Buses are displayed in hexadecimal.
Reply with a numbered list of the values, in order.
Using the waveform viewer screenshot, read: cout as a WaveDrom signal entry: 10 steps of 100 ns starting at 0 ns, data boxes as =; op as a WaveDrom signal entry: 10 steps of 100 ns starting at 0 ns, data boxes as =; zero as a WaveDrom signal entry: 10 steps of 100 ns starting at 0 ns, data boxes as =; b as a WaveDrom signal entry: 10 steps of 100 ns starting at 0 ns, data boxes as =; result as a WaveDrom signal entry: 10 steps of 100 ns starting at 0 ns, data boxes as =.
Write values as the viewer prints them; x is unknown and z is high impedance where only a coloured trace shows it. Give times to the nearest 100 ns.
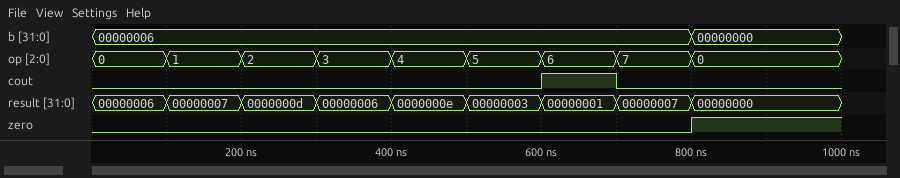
1. {name: 'cout', wave: '0.....10..'}
2. {name: 'op', wave: '=========.', data: '0 1 2 3 4 5 6 7 0'}
3. {name: 'zero', wave: '0.......1.'}
4. {name: 'b', wave: '=.......=.', data: '00000006 00000000'}
5. {name: 'result', wave: '=========.', data: '00000006 00000007 0000000d 00000006 0000000e 00000003 00000001 00000007 00000000'}
